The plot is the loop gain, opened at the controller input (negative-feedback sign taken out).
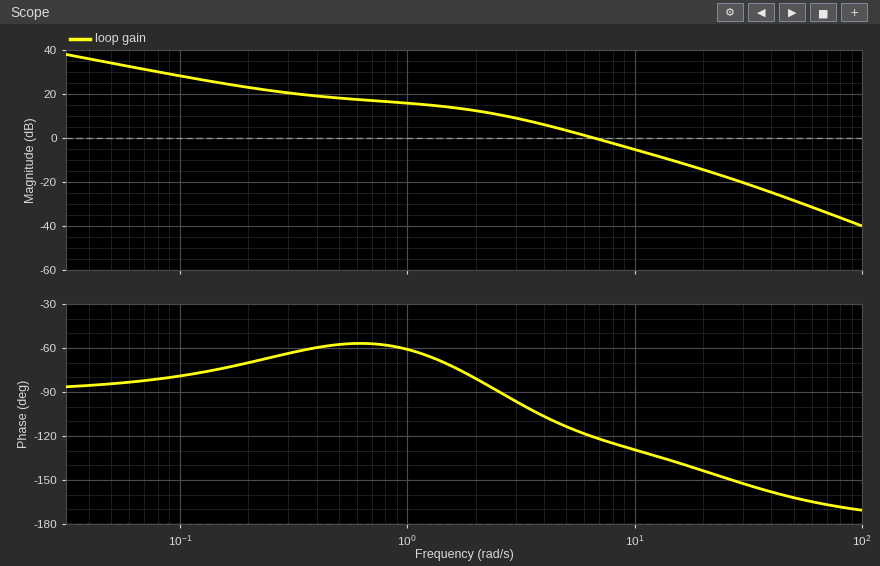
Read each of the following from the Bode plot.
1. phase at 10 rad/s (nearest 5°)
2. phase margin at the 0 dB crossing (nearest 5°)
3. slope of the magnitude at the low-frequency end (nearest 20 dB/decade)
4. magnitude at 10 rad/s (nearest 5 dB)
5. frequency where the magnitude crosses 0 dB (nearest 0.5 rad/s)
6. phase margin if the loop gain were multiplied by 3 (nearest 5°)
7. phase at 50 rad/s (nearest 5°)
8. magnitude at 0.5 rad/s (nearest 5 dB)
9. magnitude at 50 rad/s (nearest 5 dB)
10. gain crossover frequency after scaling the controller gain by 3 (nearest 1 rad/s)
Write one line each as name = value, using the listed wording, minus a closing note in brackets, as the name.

phase at 10 rad/s = -130°
phase margin at the 0 dB crossing = 60°
slope of the magnitude at the low-frequency end = -20 dB/decade
magnitude at 10 rad/s = -5 dB
frequency where the magnitude crosses 0 dB = 6.5 rad/s
phase margin if the loop gain were multiplied by 3 = 45°
phase at 50 rad/s = -160°
magnitude at 0.5 rad/s = 20 dB
magnitude at 50 rad/s = -30 dB
gain crossover frequency after scaling the controller gain by 3 = 14 rad/s
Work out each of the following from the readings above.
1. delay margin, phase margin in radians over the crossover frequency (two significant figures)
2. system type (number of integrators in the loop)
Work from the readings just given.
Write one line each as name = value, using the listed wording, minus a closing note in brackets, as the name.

delay margin, phase margin in radians over the crossover frequency = 0.16 s
system type = 1
